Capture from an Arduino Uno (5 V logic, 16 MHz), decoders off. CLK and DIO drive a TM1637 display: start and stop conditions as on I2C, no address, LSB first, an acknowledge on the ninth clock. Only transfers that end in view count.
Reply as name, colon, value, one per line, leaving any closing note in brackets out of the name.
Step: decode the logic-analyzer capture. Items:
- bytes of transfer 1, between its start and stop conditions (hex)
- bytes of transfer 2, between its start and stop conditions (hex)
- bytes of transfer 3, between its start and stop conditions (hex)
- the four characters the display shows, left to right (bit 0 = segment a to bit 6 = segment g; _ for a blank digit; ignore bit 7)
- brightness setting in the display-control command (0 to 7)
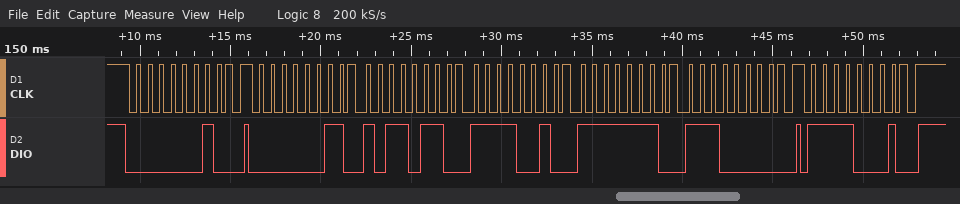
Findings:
bytes of transfer 1, between its start and stop conditions: 40
bytes of transfer 2, between its start and stop conditions: C0 6D 4F 7F 07
bytes of transfer 3, between its start and stop conditions: 8F
the four characters the display shows, left to right: 5387
brightness setting in the display-control command: 7
